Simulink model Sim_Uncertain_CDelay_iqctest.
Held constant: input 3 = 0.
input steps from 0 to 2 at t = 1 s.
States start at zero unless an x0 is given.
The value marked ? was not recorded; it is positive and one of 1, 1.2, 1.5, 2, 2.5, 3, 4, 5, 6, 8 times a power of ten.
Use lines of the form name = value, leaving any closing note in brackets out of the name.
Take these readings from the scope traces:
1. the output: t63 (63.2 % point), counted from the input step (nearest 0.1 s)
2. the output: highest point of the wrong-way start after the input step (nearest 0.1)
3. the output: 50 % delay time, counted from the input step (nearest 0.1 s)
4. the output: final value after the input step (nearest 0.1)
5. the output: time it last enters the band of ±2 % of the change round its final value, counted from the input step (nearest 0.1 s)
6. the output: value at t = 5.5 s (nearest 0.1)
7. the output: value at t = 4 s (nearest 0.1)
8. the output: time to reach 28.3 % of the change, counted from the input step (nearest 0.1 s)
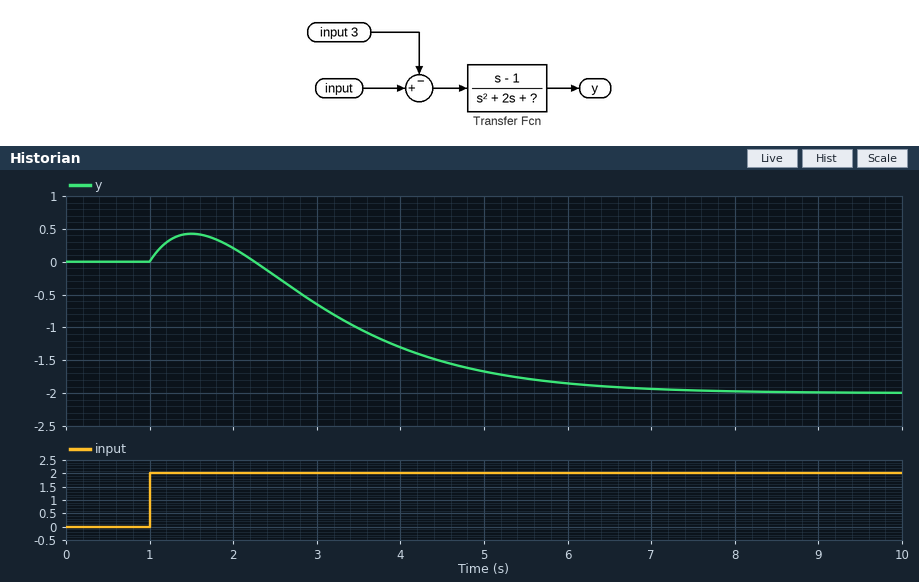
the output: t63 (63.2 % point), counted from the input step = 2.9 s
the output: highest point of the wrong-way start after the input step = 0.4
the output: 50 % delay time, counted from the input step = 2.5 s
the output: final value after the input step = -2.0
the output: time it last enters the band of ±2 % of the change round its final value, counted from the input step = 6.6 s
the output: value at t = 5.5 s = -1.8
the output: value at t = 4 s = -1.3
the output: time to reach 28.3 % of the change, counted from the input step = 1.9 s
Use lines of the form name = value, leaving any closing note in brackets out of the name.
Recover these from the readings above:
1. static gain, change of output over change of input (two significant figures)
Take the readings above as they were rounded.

static gain, change of output over change of input = -1.0
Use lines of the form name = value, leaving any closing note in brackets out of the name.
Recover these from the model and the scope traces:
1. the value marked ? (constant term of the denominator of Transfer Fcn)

the value marked ? = 1
